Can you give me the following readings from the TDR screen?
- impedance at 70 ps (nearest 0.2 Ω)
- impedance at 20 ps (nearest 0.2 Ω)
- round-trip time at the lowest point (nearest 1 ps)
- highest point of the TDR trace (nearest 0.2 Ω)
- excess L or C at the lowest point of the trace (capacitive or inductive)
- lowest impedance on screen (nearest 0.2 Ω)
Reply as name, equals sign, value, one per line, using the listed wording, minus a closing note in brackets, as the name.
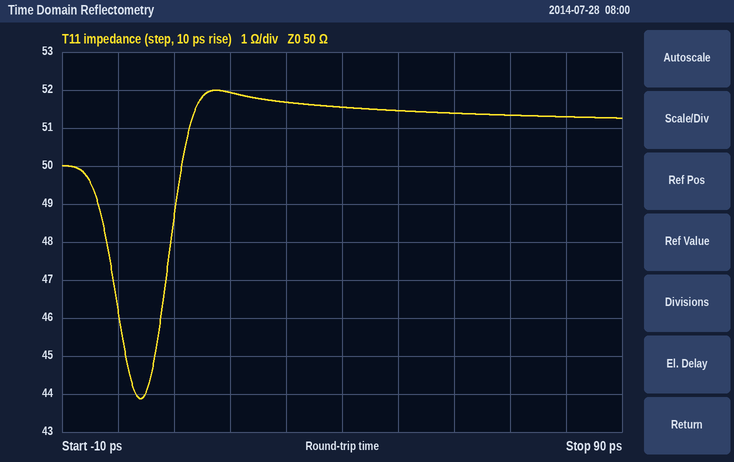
impedance at 70 ps = 51.4 Ω
impedance at 20 ps = 52.0 Ω
round-trip time at the lowest point = 4 ps
highest point of the TDR trace = 52.0 Ω
excess L or C at the lowest point of the trace = capacitive
lowest impedance on screen = 43.8 Ω
